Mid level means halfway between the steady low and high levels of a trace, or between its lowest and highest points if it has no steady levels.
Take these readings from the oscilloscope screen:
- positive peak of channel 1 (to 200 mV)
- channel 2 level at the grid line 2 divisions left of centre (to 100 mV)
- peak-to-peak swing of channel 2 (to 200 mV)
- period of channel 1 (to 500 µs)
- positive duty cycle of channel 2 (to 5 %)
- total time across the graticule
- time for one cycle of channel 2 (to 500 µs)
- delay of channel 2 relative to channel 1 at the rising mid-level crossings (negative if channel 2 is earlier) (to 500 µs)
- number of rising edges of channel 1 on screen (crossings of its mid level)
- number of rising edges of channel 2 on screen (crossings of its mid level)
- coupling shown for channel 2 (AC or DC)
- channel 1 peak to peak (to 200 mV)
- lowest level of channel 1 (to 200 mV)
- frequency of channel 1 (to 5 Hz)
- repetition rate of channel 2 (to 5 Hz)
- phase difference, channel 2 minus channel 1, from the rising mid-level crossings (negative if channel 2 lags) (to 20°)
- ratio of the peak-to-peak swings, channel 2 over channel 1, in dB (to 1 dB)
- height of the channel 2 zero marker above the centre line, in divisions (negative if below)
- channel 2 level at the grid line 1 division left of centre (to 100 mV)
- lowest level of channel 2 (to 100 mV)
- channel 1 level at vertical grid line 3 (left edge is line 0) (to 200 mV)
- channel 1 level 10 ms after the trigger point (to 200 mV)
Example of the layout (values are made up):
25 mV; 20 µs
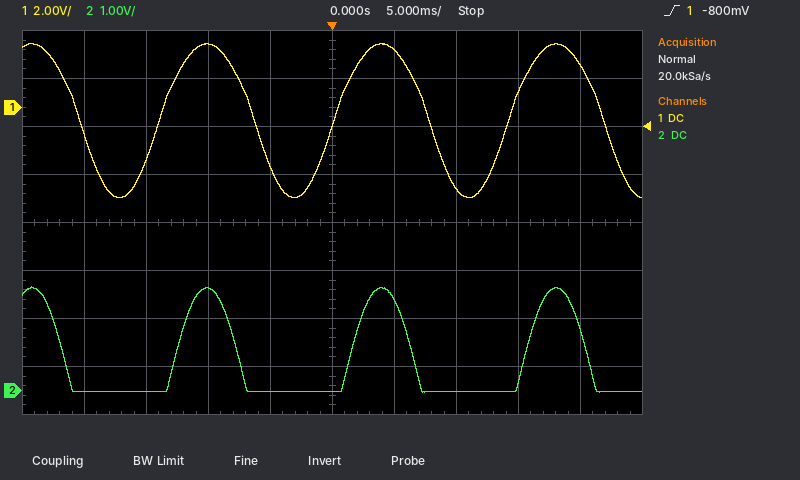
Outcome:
2.6 V; 2.1 V; 2.2 V; 14.0 ms; 30 %; 50 ms; 14.0 ms; +1.5 ms; 3; 3; DC; 6.4 V; -3.8 V; 70 Hz; 70 Hz; -40°; -9 dB; -3.5 div; 0.0 V; 0.0 V; 2.6 V; -3.4 V
